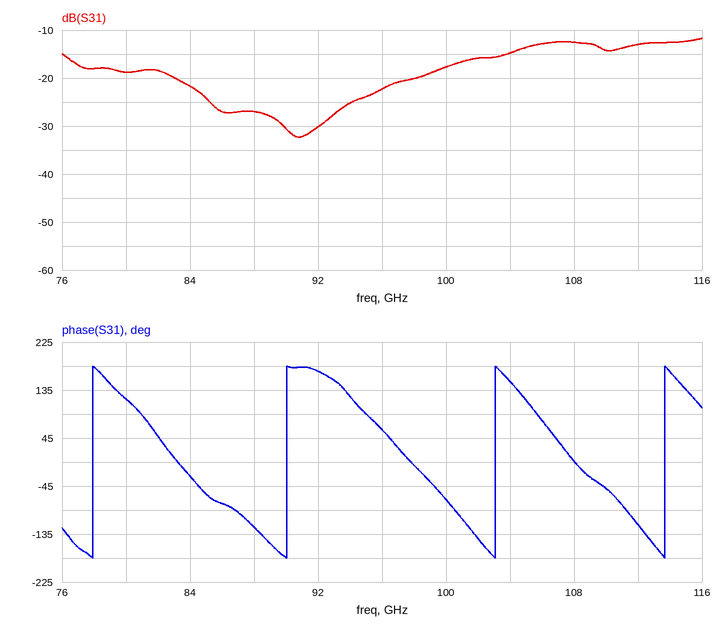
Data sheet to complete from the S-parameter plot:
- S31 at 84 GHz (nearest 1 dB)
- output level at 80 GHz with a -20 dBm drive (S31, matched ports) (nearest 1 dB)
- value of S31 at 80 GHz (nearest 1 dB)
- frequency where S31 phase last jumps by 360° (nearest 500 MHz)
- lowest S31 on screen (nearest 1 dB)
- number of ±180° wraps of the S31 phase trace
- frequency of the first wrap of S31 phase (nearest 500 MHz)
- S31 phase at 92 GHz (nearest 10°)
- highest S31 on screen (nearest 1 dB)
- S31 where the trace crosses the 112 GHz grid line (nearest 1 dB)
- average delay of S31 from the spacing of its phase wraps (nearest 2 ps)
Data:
-22 dB
-39 dBm
-19 dB
113.5 GHz
-32 dB
4
78.0 GHz
170°
-12 dB
-13 dB
84 ps
